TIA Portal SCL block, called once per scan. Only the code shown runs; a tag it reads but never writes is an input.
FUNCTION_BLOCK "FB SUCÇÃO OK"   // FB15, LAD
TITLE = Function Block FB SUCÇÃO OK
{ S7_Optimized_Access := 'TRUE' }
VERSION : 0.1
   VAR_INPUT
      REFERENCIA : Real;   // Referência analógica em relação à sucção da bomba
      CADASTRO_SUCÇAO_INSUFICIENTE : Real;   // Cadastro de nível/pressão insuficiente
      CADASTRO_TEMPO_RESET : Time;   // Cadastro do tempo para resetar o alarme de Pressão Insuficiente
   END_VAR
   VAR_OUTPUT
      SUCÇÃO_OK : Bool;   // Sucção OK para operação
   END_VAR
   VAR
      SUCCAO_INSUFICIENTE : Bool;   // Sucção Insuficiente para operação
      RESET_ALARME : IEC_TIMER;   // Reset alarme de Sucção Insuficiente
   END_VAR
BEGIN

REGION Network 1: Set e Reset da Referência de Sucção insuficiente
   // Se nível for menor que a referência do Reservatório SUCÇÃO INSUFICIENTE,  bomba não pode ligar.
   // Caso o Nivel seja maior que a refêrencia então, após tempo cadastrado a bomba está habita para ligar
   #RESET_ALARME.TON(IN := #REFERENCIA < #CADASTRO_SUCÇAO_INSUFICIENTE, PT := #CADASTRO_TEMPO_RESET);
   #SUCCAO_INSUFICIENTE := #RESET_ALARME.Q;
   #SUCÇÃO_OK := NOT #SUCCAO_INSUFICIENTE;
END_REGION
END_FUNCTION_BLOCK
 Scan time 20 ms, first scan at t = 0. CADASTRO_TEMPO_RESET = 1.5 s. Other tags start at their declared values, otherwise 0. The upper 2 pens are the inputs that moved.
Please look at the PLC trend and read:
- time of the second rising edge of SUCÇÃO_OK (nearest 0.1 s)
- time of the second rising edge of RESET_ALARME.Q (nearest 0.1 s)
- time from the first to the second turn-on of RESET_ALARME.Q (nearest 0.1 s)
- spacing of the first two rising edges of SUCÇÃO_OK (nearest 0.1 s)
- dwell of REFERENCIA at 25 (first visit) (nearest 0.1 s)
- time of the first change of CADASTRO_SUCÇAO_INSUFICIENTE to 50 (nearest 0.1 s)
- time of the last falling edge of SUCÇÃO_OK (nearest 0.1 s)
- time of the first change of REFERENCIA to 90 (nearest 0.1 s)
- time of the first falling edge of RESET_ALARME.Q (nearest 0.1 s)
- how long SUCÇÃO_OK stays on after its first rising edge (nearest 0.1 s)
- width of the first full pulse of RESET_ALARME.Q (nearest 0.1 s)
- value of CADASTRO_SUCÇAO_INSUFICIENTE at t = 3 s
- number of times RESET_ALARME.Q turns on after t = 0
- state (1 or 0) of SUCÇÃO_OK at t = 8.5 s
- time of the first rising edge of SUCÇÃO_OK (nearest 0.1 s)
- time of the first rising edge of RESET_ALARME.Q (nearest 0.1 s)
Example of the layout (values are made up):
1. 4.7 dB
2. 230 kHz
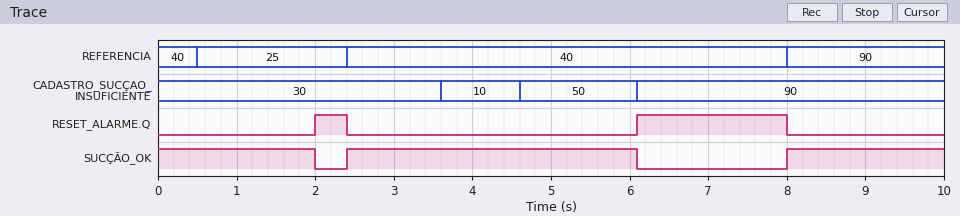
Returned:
1. 8.0 s
2. 6.1 s
3. 4.1 s
4. 5.6 s
5. 1.9 s
6. 4.6 s
7. 6.1 s
8. 8.0 s
9. 2.4 s
10. 3.7 s
11. 0.4 s
12. 30
13. 2
14. 1
15. 2.4 s
16. 2.0 s
